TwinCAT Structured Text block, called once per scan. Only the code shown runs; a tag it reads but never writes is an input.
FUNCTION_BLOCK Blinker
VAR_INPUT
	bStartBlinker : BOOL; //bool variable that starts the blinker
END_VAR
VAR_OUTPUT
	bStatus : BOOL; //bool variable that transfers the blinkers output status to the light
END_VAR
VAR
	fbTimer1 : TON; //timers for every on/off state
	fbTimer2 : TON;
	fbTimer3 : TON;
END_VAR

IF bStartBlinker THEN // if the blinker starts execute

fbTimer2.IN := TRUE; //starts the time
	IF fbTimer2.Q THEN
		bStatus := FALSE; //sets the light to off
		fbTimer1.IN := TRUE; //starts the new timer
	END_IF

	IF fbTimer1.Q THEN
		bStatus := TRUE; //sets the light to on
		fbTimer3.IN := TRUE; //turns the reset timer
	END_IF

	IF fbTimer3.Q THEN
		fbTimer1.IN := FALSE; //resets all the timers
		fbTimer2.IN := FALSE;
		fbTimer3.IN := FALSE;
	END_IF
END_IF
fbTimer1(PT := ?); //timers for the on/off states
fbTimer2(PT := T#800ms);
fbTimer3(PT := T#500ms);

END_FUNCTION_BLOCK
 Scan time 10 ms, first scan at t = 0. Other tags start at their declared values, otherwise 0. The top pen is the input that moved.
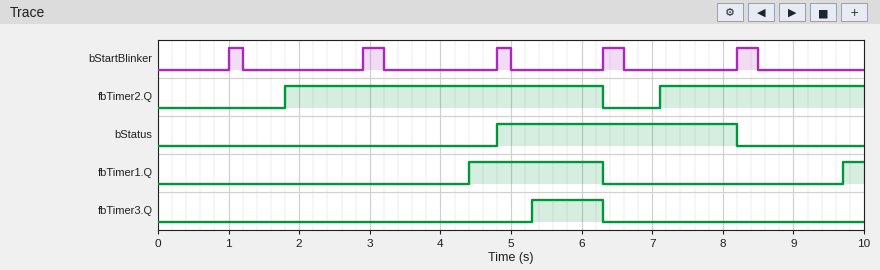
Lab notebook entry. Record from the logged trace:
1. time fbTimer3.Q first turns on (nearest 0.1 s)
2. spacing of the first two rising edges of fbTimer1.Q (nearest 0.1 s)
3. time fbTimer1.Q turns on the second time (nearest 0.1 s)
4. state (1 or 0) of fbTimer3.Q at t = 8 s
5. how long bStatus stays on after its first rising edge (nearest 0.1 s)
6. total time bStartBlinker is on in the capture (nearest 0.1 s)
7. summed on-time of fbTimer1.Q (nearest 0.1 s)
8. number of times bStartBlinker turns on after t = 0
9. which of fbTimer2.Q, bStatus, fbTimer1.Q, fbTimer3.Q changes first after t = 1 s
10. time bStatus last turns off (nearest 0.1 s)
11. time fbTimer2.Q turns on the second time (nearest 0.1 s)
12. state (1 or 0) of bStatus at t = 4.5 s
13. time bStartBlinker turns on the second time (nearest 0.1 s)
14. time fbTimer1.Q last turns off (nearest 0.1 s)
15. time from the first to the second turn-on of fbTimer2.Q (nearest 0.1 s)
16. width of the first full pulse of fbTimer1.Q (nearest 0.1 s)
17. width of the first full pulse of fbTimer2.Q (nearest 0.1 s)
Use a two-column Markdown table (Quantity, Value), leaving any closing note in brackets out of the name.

| Quantity | Value |
|---|---|
| time fbTimer3.Q first turns on | 5.3 s |
| spacing of the first two rising edges of fbTimer1.Q | 5.3 s |
| time fbTimer1.Q turns on the second time | 9.7 s |
| state (1 or 0) of fbTimer3.Q at t = 8 s | 0 |
| how long bStatus stays on after its first rising edge | 3.4 s |
| total time bStartBlinker is on in the capture | 1.3 s |
| summed on-time of fbTimer1.Q | 2.2 s |
| number of times bStartBlinker turns on after t = 0 | 5 |
| which of fbTimer2.Q, bStatus, fbTimer1.Q, fbTimer3.Q changes first after t = 1 s | fbTimer2.Q |
| time bStatus last turns off | 8.2 s |
| time fbTimer2.Q turns on the second time | 7.1 s |
| state (1 or 0) of bStatus at t = 4.5 s | 0 |
| time bStartBlinker turns on the second time | 2.9 s |
| time fbTimer1.Q last turns off | 6.3 s |
| time from the first to the second turn-on of fbTimer2.Q | 5.3 s |
| width of the first full pulse of fbTimer1.Q | 1.9 s |
| width of the first full pulse of fbTimer2.Q | 4.5 s |
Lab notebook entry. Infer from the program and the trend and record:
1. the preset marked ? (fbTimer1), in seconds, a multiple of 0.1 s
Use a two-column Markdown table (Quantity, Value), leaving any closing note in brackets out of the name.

| Quantity | Value |
|---|---|
| the preset marked ? (fbTimer1), in seconds, a multiple of 0.1 s | 1.5 s |
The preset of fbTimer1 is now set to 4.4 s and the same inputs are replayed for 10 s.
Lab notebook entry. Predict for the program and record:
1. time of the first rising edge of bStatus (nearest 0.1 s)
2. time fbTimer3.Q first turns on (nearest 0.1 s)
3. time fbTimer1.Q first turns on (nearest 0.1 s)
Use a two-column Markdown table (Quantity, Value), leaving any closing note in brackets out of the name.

| Quantity | Value |
|---|---|
| time of the first rising edge of bStatus | 8.2 s |
| time fbTimer3.Q first turns on | 8.7 s |
| time fbTimer1.Q first turns on | 7.3 s |
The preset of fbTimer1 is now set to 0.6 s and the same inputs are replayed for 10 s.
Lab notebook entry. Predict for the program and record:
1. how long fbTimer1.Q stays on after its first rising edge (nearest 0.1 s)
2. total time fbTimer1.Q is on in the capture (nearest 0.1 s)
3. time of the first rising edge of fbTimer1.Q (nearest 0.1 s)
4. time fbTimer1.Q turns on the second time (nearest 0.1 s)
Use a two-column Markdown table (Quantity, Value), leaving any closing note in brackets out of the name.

| Quantity | Value |
|---|---|
| how long fbTimer1.Q stays on after its first rising edge | 2.8 s |
| total time fbTimer1.Q is on in the capture | 4.0 s |
| time of the first rising edge of fbTimer1.Q | 3.5 s |
| time fbTimer1.Q turns on the second time | 8.8 s |
